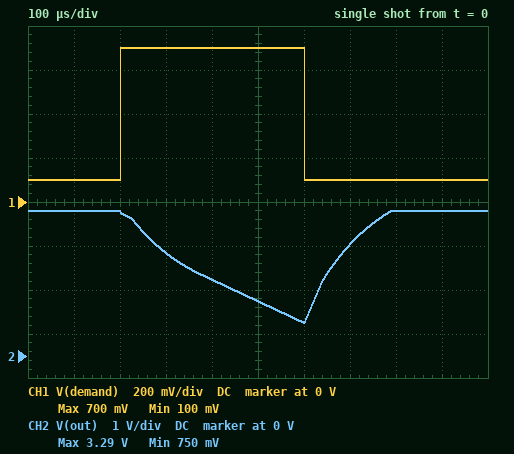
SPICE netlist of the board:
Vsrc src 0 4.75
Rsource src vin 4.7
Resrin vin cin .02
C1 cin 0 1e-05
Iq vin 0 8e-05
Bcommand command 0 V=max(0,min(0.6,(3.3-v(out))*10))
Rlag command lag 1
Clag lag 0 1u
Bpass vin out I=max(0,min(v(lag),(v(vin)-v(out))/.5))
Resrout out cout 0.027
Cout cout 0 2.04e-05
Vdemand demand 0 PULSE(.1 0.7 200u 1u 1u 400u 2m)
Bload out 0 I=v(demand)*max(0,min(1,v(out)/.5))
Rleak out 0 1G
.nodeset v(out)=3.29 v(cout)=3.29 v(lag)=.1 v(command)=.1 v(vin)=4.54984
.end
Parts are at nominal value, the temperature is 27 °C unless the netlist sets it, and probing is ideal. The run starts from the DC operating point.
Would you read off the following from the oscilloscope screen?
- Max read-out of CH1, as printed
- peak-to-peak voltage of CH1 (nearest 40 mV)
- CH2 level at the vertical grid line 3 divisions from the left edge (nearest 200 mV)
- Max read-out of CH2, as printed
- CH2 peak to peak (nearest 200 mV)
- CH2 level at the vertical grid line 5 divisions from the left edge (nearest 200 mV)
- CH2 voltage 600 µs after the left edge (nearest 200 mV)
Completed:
700 mV
600 mV
2.4 V
3.29 V
2.6 V
1.2 V
800 mV
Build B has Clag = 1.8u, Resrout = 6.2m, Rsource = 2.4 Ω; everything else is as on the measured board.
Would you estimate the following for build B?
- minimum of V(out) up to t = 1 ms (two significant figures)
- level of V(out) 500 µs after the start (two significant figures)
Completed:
1.3 V
1.8 V
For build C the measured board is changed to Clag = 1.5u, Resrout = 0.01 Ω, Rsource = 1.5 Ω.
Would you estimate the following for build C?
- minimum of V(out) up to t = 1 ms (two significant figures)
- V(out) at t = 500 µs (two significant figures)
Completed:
1.3 V
1.8 V
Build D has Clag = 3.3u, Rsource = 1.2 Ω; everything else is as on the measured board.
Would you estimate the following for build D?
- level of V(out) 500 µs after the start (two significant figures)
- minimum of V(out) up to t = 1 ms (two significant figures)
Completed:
1.7 V
1.2 V
